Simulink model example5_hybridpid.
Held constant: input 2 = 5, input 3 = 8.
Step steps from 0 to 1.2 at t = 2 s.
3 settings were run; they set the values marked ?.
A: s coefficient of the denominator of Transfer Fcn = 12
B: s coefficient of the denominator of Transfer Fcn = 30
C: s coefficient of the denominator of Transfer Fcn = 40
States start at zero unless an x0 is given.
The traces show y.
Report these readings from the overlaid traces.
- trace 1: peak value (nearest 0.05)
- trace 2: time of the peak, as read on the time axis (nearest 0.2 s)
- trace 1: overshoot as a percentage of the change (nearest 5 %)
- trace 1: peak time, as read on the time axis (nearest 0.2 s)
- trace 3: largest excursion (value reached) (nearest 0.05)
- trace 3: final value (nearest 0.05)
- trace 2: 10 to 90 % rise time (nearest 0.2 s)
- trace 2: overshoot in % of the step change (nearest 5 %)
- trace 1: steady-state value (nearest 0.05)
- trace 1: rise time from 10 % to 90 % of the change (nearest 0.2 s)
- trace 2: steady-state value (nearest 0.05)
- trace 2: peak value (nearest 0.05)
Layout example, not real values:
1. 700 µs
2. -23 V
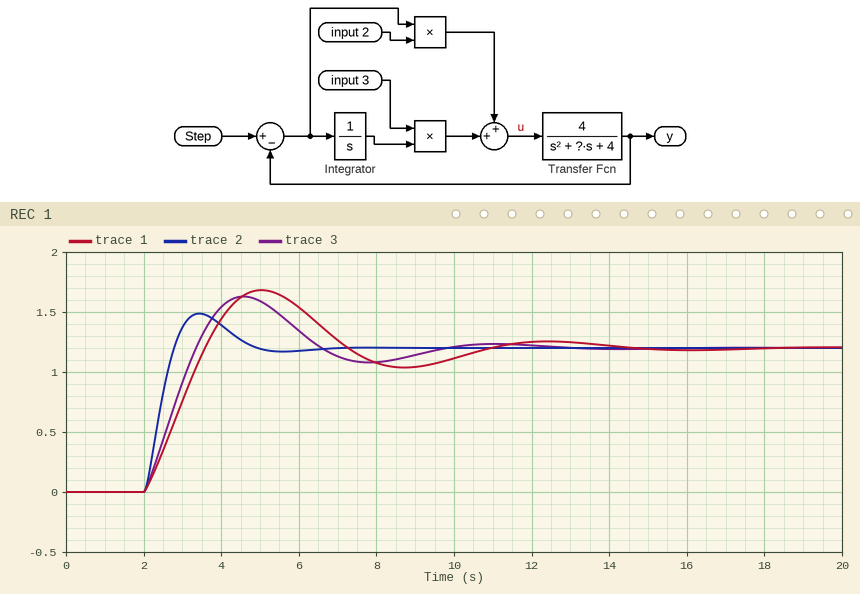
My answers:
1. 1.70
2. 3.4 s
3. 40 %
4. 5.0 s
5. 1.65
6. 1.20
7. 0.6 s
8. 25 %
9. 1.20
10. 1.2 s
11. 1.20
12. 1.50
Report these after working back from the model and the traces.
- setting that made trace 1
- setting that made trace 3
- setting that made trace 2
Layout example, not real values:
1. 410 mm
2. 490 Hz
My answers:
1. C
2. B
3. A
